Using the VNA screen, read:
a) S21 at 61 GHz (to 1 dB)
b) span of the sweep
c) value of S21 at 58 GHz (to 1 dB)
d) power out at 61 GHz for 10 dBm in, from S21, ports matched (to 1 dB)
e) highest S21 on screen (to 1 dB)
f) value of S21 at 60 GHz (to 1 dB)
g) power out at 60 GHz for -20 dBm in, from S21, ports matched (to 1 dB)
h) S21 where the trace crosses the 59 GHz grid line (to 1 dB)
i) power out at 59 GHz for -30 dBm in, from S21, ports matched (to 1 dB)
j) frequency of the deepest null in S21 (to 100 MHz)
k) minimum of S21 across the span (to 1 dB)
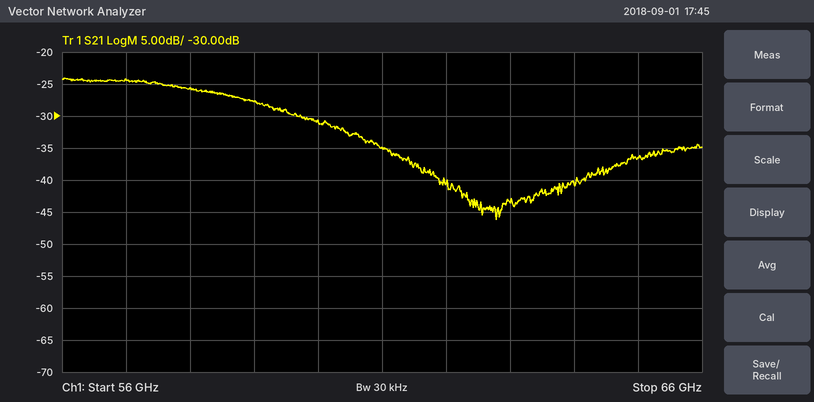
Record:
-35 dB
10 GHz
-26 dB
-25 dBm
-24 dB
-31 dB
-51 dBm
-28 dB
-58 dBm
62.8 GHz
-46 dB
